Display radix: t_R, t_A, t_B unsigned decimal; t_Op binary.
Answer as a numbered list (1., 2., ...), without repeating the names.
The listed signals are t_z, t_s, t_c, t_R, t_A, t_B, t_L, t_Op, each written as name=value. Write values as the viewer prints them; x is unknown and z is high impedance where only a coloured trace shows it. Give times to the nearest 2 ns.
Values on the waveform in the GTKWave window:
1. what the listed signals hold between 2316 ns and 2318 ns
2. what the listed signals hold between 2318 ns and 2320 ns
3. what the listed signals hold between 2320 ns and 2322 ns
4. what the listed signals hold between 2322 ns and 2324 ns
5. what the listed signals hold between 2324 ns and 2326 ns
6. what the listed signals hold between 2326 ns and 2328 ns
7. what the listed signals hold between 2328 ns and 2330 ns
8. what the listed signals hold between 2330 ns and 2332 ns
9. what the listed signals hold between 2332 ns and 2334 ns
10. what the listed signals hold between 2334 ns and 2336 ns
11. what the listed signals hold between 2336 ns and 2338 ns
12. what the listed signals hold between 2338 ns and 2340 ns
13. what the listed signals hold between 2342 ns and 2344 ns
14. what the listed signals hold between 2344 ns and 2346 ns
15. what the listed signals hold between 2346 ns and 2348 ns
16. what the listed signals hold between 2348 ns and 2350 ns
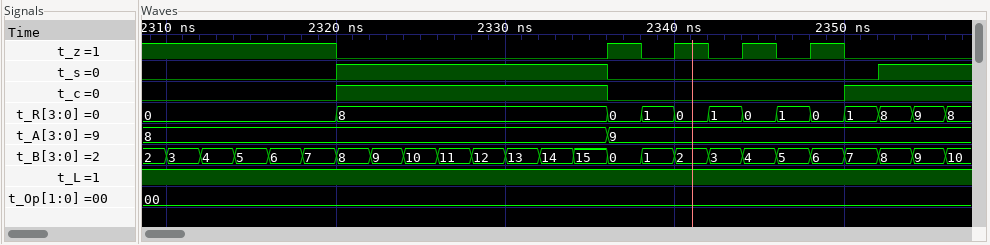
1. t_z=1, t_s=0, t_c=0, t_R=0, t_A=8, t_B=6, t_L=1, t_Op=00
2. t_z=1, t_s=0, t_c=0, t_R=0, t_A=8, t_B=7, t_L=1, t_Op=00
3. t_z=0, t_s=1, t_c=1, t_R=8, t_A=8, t_B=8, t_L=1, t_Op=00
4. t_z=0, t_s=1, t_c=1, t_R=8, t_A=8, t_B=9, t_L=1, t_Op=00
5. t_z=0, t_s=1, t_c=1, t_R=8, t_A=8, t_B=10, t_L=1, t_Op=00
6. t_z=0, t_s=1, t_c=1, t_R=8, t_A=8, t_B=11, t_L=1, t_Op=00
7. t_z=0, t_s=1, t_c=1, t_R=8, t_A=8, t_B=12, t_L=1, t_Op=00
8. t_z=0, t_s=1, t_c=1, t_R=8, t_A=8, t_B=13, t_L=1, t_Op=00
9. t_z=0, t_s=1, t_c=1, t_R=8, t_A=8, t_B=14, t_L=1, t_Op=00
10. t_z=0, t_s=1, t_c=1, t_R=8, t_A=8, t_B=15, t_L=1, t_Op=00
11. t_z=1, t_s=0, t_c=0, t_R=0, t_A=9, t_B=0, t_L=1, t_Op=00
12. t_z=0, t_s=0, t_c=0, t_R=1, t_A=9, t_B=1, t_L=1, t_Op=00
13. t_z=0, t_s=0, t_c=0, t_R=1, t_A=9, t_B=3, t_L=1, t_Op=00
14. t_z=1, t_s=0, t_c=0, t_R=0, t_A=9, t_B=4, t_L=1, t_Op=00
15. t_z=0, t_s=0, t_c=0, t_R=1, t_A=9, t_B=5, t_L=1, t_Op=00
16. t_z=1, t_s=0, t_c=0, t_R=0, t_A=9, t_B=6, t_L=1, t_Op=00
